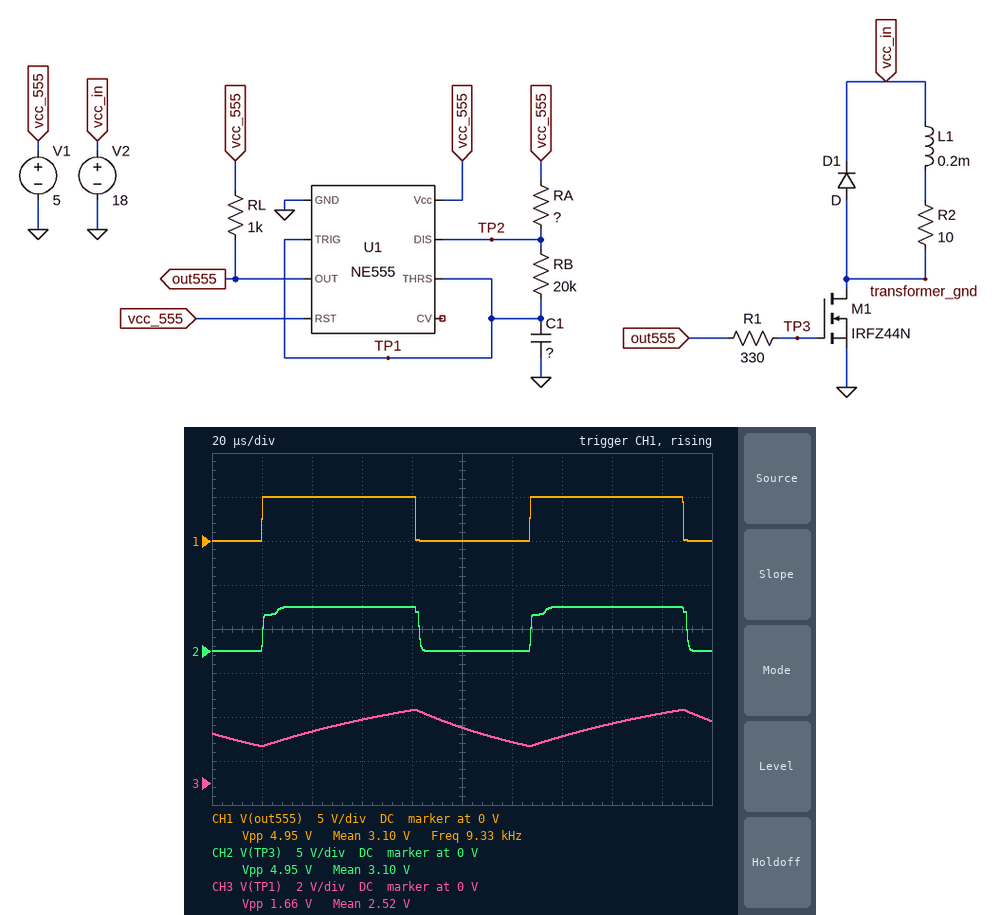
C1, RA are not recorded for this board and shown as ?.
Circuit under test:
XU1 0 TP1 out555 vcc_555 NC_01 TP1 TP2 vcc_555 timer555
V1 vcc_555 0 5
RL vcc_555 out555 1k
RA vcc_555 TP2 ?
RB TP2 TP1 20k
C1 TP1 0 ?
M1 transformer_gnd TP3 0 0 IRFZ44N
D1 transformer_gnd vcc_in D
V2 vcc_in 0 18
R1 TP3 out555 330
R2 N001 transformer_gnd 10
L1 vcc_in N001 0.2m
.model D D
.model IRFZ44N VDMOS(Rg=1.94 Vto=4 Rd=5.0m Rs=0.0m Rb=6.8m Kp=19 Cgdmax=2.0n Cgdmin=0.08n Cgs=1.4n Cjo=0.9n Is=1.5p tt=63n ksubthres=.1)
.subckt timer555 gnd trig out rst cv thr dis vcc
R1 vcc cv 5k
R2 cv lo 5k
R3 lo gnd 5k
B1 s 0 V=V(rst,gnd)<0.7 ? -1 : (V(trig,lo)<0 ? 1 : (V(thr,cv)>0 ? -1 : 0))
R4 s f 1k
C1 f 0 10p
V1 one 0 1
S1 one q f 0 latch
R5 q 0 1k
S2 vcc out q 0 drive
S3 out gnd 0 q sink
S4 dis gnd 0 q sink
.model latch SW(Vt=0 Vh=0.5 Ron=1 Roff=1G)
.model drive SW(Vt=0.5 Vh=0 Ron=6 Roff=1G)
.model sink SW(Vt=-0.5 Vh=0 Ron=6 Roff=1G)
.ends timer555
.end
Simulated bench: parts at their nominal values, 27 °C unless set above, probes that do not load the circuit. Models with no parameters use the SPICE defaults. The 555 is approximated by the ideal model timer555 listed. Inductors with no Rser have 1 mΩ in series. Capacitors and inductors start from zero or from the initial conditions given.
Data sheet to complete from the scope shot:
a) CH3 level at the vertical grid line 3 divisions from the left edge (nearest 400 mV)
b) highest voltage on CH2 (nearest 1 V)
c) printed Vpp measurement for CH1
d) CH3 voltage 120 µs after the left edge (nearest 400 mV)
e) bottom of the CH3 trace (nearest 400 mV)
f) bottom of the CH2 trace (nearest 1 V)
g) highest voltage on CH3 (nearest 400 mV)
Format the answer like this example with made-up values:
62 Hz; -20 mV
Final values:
2.8 V; 5 V; 4.95 V; 2.0 V; 1.6 V; 0 V; 3.2 V
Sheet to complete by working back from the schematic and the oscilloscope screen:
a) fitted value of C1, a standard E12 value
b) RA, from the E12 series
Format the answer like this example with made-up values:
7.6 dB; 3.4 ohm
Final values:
3.3 nF; 6.8 kΩ
